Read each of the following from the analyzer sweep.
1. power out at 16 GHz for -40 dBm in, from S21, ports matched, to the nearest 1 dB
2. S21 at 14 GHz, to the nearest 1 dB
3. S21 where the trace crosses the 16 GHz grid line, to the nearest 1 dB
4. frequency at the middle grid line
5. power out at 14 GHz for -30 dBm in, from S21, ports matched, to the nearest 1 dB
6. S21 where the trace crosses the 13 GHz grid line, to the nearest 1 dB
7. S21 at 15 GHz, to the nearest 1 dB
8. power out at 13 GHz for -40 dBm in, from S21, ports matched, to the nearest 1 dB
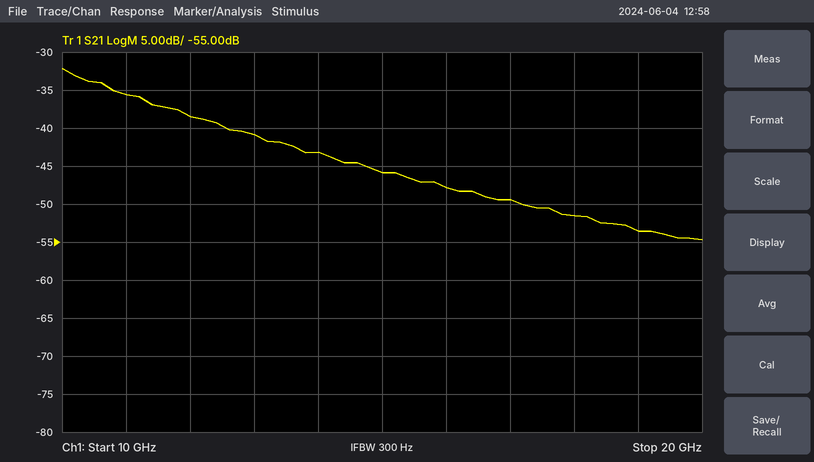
-88 dBm
-43 dB
-48 dB
15 GHz
-73 dBm
-41 dB
-46 dB
-81 dBm
